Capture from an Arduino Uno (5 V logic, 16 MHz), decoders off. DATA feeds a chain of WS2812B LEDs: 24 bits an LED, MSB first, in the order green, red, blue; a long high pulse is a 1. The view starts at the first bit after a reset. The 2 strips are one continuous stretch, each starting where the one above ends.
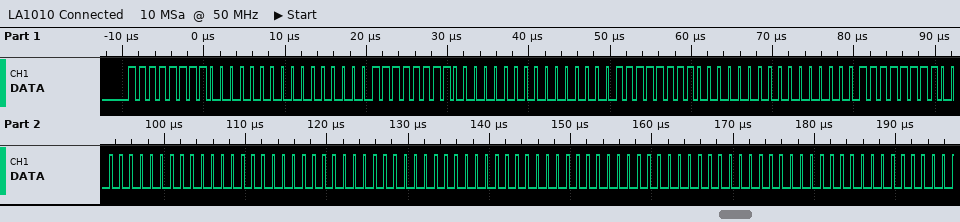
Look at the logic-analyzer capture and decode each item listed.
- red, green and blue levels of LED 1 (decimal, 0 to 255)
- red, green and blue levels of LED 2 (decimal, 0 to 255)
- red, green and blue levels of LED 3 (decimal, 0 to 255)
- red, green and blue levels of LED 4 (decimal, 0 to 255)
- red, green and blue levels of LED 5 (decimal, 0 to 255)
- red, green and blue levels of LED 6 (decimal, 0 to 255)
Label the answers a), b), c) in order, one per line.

a) 0, 255, 0
b) 0, 255, 0
c) 0, 255, 0
d) 0, 255, 0
e) 0, 0, 0
f) 0, 0, 0
